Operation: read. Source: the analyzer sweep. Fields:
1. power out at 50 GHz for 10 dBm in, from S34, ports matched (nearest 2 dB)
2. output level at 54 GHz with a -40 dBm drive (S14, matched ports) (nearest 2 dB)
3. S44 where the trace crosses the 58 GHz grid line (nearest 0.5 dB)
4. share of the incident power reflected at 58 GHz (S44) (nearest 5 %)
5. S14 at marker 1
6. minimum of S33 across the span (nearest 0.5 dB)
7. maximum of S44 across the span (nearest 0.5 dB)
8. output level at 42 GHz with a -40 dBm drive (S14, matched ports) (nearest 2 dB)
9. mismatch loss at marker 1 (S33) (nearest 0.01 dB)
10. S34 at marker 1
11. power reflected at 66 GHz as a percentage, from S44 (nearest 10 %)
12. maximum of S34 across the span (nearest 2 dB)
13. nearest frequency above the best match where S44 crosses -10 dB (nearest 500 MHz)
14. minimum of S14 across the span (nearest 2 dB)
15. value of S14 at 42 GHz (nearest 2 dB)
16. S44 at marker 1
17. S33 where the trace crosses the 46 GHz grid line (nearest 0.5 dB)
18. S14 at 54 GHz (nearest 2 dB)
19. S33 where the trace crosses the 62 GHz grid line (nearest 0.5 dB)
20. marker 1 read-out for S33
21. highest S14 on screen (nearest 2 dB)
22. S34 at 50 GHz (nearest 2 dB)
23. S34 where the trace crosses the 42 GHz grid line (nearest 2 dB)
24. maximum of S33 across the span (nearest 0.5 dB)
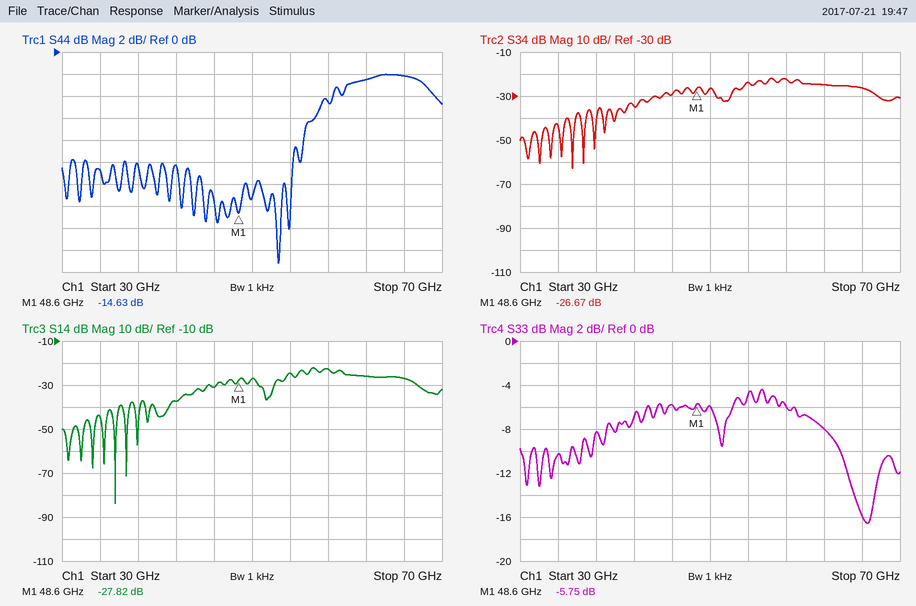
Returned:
-16 dBm
-64 dBm
-4.5 dB
35 %
-27.82 dB
-16.5 dB
-2.0 dB
-78 dBm
1.34 dB
-26.67 dB
60 %
-22 dB
54.5 GHz
-84 dB
-38 dB
-14.63 dB
-6.0 dB
-24 dB
-8.0 dB
-5.75 dB
-22 dB
-26 dB
-34 dB
-4.5 dB
